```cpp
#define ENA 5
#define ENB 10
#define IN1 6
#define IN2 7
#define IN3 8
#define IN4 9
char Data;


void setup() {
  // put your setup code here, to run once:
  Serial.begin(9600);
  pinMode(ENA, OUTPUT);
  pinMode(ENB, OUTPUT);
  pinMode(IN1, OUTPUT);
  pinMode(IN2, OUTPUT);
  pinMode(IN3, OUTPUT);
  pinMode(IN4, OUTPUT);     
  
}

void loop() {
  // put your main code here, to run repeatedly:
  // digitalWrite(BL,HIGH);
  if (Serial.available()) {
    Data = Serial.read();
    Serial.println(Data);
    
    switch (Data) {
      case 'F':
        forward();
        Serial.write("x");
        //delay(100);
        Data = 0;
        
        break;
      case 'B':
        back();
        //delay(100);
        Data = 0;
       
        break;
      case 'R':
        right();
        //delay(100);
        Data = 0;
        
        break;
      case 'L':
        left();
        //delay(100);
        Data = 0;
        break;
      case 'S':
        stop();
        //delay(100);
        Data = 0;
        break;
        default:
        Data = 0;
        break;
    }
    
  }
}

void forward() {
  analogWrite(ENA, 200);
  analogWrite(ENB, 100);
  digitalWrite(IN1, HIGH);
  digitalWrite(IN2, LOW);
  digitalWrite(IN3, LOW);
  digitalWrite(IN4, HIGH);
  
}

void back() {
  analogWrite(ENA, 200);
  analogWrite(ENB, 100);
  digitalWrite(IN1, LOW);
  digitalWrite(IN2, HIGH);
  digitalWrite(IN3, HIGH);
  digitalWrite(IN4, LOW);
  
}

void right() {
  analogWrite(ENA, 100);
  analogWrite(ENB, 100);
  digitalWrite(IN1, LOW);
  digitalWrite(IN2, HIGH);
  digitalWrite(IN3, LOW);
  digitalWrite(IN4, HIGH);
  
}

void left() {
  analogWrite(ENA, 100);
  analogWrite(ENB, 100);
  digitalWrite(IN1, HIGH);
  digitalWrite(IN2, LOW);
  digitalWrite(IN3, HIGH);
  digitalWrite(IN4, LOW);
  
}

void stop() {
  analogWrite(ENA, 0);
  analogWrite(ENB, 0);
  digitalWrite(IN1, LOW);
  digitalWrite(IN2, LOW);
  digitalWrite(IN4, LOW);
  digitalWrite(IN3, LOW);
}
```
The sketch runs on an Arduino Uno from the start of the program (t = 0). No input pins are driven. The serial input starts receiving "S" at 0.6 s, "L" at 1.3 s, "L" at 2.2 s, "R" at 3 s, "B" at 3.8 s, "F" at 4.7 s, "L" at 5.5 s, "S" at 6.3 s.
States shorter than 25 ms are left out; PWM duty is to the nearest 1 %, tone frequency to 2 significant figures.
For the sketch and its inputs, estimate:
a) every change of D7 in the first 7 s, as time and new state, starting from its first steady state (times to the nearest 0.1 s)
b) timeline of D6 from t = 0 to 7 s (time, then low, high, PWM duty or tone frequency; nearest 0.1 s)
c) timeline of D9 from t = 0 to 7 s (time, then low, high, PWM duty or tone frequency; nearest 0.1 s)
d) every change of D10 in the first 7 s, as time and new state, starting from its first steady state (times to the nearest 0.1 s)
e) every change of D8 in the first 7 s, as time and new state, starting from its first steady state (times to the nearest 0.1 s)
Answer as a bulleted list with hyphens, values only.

- 0 s low; 3 s high; 4.7 s low
- 0 s low; 1.3 s high; 3 s low; 4.7 s high; 6.3 s low
- 0 s low; 3 s high; 3.8 s low; 4.7 s high; 5.5 s low
- 0 s low; 1.3 s PWM 39 %; 6.3 s low
- 0 s low; 1.3 s high; 3 s low; 3.8 s high; 4.7 s low; 5.5 s high; 6.3 s low
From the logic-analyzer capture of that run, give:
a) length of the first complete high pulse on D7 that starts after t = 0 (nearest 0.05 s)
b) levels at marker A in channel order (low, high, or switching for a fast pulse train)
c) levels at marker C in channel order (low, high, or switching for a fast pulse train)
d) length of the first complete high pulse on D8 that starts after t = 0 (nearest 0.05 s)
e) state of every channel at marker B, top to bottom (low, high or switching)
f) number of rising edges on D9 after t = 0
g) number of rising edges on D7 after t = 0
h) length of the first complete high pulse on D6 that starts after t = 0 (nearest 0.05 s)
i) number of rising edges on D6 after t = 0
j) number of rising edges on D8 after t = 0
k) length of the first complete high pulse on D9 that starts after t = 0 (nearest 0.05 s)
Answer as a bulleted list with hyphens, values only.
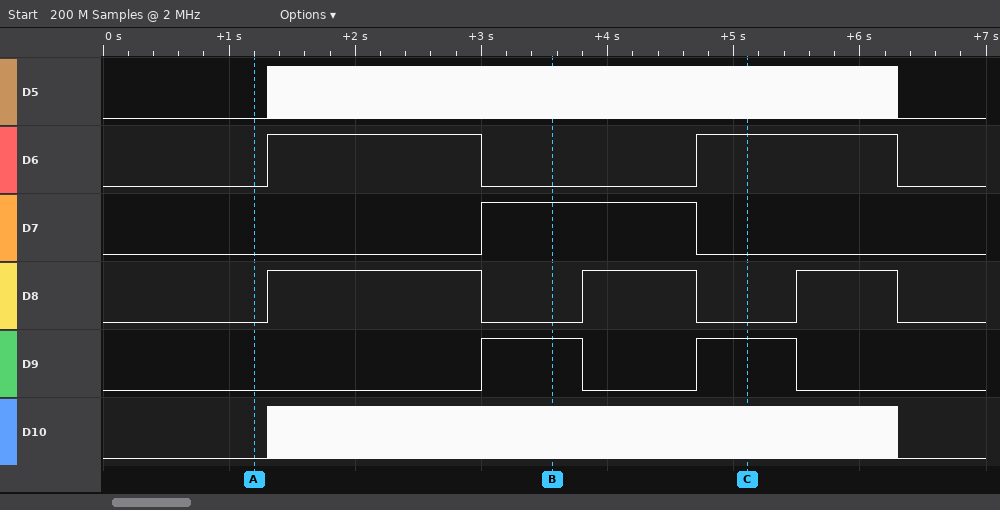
- 1.70 s
- D5 low, D6 low, D7 low, D8 low, D9 low, D10 low
- D5 switching, D6 high, D7 low, D8 low, D9 high, D10 switching
- 1.70 s
- D5 switching, D6 low, D7 high, D8 low, D9 high, D10 switching
- 2
- 1
- 1.70 s
- 2
- 3
- 0.80 s
